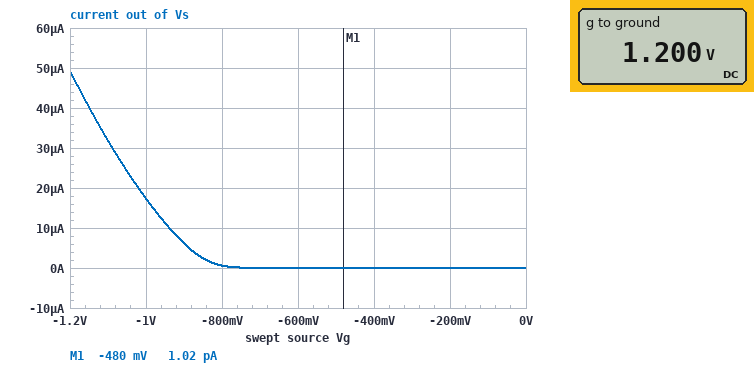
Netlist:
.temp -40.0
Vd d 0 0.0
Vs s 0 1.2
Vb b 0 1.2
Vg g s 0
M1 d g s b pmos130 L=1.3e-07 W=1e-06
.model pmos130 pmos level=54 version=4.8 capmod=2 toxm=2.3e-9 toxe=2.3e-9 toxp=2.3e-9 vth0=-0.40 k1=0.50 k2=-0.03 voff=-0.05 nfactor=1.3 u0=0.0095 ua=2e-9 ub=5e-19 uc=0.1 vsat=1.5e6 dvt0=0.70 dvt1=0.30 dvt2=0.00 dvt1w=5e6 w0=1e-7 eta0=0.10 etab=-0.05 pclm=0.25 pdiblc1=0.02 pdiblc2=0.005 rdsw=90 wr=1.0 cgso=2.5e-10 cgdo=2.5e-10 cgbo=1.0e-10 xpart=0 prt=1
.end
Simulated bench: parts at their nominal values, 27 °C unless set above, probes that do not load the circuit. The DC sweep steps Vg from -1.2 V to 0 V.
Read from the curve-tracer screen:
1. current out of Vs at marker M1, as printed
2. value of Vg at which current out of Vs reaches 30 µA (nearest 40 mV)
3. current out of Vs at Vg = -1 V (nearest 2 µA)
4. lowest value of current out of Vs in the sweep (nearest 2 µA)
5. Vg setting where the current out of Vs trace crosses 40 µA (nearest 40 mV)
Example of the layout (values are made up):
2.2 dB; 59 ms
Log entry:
1.02 pA; -1.08 V; 18 µA; 0 A; -1.16 V
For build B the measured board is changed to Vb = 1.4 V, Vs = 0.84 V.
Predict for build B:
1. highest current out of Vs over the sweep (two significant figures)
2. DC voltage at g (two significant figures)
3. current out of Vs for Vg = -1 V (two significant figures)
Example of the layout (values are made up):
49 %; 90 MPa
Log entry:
770 µA; 840 mV; 150 µA
